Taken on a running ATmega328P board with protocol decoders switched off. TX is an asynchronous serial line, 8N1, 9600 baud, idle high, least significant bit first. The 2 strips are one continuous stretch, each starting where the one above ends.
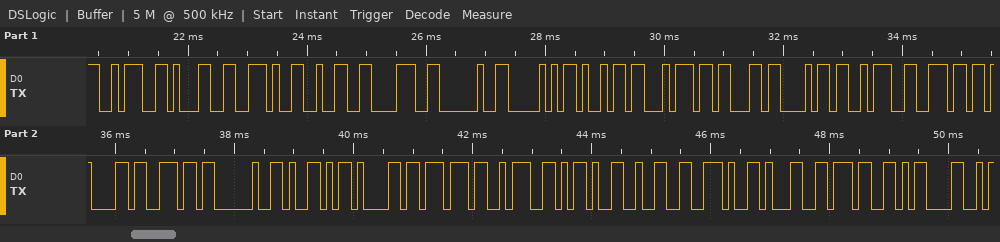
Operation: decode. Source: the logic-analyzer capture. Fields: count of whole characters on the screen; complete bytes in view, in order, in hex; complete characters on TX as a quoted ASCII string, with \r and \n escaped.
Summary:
26
0x3A 0x31 0x2E 0x32 0x38 0x20 0x50 0x69 0x74 0x63 0x68 0x3A 0x6E 0x61 0x6E 0x20 0x59 0x61 0x77 0x3A 0x2D 0x32 0x2E 0x31 0x37 0x0D
":1.28 Pitch:nan Yaw:-2.17\r"
